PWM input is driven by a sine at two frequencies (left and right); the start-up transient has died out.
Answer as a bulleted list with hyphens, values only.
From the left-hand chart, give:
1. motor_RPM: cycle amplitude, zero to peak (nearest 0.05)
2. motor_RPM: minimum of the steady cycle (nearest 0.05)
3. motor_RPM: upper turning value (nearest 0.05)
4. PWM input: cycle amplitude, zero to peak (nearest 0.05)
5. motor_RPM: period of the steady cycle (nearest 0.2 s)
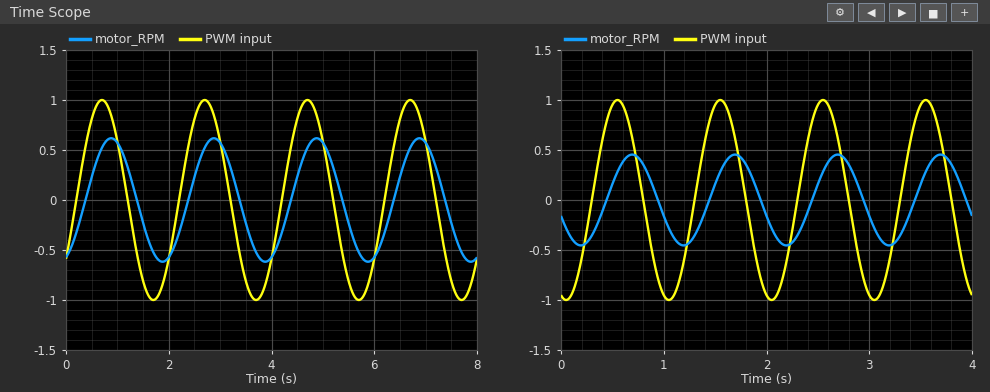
- 0.60
- -0.60
- 0.60
- 1.00
- 2.0 s
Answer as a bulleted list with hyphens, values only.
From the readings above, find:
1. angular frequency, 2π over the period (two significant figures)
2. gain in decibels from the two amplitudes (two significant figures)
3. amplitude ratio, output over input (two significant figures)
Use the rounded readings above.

- 3.1 rad/s
- -4.4 dB
- 0.60
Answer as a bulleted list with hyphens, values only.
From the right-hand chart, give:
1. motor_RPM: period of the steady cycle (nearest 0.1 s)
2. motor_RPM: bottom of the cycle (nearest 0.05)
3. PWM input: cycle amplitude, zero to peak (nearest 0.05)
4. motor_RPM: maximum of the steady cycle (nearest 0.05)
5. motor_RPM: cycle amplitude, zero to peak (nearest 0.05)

- 1.0 s
- -0.45
- 1.00
- 0.45
- 0.45
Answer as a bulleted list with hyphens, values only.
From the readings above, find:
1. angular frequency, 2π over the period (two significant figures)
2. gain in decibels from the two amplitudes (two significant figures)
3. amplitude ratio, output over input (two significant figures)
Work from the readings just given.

- 6.3 rad/s
- -6.9 dB
- 0.45
